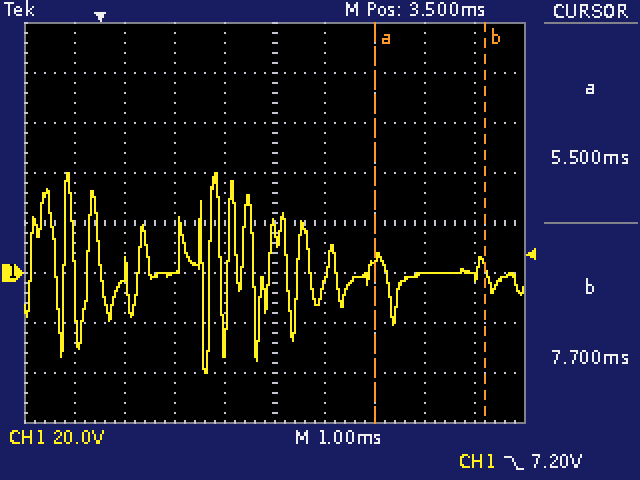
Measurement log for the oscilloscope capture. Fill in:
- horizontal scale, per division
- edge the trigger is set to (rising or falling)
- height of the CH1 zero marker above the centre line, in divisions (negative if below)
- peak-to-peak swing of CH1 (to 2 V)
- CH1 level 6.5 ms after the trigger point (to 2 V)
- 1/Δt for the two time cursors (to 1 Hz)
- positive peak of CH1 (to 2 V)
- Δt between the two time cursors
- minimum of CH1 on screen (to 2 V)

1 ms
falling
-1.0 div
80 V
0 V
455 Hz
40 V
2.2 ms
-40 V
